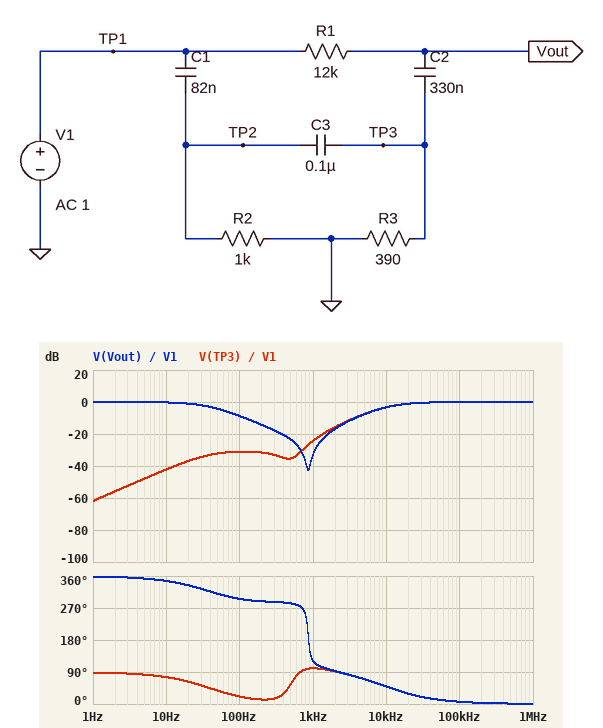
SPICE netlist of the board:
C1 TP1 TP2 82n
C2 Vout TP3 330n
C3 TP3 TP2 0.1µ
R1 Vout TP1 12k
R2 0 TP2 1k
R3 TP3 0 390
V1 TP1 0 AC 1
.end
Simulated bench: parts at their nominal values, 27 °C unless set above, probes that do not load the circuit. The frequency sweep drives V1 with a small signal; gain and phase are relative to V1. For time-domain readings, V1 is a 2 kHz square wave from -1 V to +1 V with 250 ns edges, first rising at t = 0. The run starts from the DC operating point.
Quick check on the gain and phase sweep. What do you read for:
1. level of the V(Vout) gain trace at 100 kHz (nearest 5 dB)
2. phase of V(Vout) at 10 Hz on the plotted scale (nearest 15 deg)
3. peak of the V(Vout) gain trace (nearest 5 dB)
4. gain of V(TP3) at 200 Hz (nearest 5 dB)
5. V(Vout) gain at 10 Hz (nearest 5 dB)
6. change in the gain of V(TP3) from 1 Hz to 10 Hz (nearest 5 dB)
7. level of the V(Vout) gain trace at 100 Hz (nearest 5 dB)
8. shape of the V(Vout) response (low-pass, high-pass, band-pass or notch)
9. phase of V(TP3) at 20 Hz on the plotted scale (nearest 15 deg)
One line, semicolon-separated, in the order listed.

0 dB; 345 deg; 0 dB; -30 dB; 0 dB; 20 dB; -10 dB; notch; 60 deg
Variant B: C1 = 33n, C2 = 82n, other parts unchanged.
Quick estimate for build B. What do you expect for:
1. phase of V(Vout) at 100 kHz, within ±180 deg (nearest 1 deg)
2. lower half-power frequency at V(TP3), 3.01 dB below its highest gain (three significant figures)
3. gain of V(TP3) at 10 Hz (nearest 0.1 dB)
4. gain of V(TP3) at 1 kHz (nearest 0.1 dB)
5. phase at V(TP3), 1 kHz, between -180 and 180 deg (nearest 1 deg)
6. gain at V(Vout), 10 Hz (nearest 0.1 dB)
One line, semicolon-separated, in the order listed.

12 deg; 20.9 kHz; -54.0 dB; -31.5 dB; 78 deg; 0 dB
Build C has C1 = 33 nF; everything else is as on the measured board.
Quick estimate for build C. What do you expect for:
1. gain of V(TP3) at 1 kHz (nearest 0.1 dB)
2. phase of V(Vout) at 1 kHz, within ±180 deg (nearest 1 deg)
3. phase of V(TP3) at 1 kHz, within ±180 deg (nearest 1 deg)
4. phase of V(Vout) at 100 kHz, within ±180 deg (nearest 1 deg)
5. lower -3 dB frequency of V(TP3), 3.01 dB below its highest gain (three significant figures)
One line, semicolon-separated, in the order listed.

-32.7 dB; -70 deg; 76 deg; 12 deg; 20.9 kHz
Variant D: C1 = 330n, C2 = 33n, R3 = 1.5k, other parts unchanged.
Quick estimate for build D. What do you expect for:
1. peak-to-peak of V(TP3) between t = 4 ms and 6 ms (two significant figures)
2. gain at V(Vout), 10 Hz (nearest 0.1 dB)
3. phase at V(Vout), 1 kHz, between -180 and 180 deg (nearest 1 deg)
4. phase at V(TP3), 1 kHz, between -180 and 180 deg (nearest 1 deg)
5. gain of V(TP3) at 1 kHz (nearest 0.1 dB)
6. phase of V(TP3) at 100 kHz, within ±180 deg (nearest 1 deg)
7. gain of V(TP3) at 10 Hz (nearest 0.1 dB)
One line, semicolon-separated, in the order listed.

3.9 V; 0 dB; 35 deg; 67 deg; -6.3 dB; 1 deg; -50.1 dB
